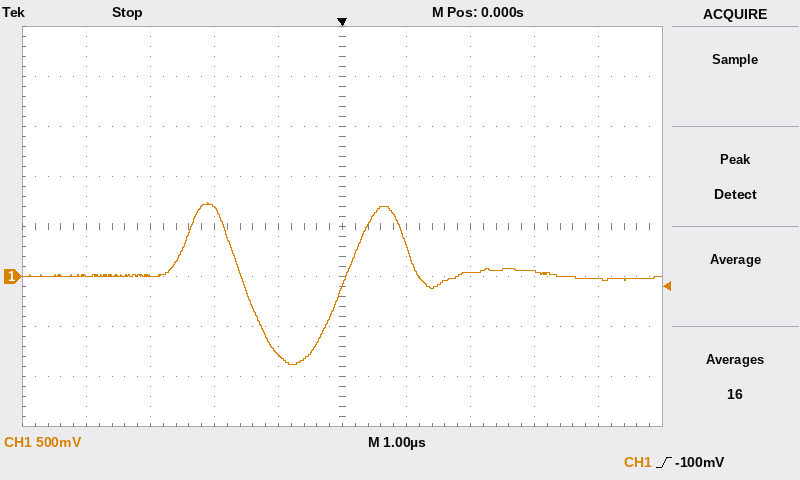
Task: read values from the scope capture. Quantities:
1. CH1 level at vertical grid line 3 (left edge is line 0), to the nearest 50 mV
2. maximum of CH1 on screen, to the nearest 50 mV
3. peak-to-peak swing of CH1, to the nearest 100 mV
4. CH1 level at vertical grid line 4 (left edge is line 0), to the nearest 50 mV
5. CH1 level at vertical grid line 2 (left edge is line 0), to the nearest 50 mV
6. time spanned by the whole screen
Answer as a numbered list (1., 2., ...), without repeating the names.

1. 700 mV
2. 750 mV
3. 1.60 V
4. -800 mV
5. 0 mV
6. 10 µs
